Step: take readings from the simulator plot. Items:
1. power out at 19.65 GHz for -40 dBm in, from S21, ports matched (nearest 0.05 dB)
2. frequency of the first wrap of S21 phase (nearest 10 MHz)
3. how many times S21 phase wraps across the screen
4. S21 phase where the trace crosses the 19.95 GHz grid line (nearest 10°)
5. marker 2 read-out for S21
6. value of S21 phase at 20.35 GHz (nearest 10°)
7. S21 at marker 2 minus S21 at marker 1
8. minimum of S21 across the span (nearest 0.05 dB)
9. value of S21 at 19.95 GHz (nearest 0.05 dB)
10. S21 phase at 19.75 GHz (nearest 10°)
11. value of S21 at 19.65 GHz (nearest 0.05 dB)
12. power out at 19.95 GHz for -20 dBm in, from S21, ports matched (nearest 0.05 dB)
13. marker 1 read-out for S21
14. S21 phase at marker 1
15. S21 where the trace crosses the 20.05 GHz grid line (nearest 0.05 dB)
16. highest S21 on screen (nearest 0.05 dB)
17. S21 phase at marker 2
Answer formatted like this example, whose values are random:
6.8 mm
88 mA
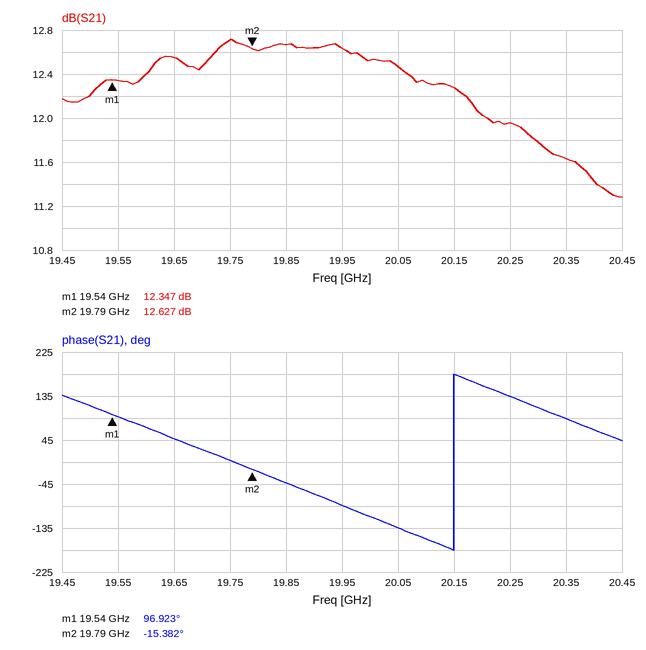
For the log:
-27.45 dBm
20.15 GHz
1
-90°
12.627 dB
90°
0.280 dB
11.30 dB
12.65 dB
0°
12.55 dB
-7.35 dBm
12.347 dB
96.923°
12.45 dB
12.70 dB
-15.382°
